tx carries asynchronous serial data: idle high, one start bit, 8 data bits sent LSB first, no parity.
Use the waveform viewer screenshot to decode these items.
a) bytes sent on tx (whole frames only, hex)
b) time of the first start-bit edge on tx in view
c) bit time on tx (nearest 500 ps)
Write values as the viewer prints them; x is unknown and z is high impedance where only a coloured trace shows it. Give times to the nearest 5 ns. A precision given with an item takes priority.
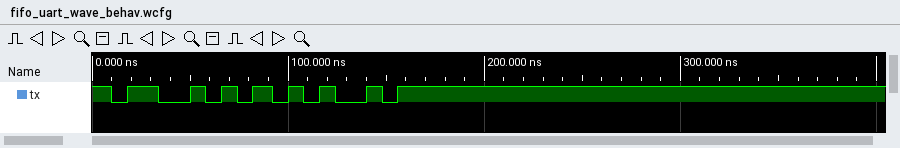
53, A5
10 ns
8000 ps
